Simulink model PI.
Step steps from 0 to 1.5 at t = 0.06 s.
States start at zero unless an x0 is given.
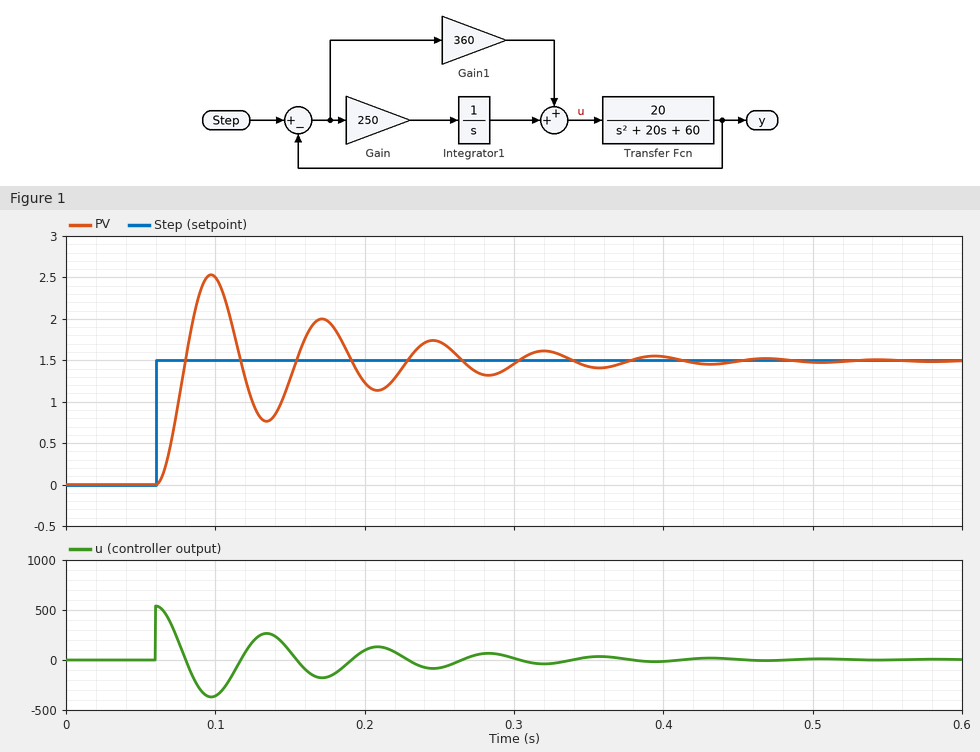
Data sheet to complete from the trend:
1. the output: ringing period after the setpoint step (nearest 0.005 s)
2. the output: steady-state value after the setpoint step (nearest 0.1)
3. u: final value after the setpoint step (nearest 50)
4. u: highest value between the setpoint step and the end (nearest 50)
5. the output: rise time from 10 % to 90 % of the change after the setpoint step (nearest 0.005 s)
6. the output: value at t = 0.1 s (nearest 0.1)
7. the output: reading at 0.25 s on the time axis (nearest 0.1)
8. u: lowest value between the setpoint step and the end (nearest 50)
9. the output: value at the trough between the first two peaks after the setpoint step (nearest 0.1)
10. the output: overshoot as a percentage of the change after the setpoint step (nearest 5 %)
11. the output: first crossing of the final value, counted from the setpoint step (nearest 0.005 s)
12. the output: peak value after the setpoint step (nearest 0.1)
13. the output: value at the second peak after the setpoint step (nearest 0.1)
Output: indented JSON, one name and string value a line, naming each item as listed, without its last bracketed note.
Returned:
{
  "the output: ringing period after the setpoint step": "0.075 s",
  "the output: steady-state value after the setpoint step": "1.5",
  "u: final value after the setpoint step": "0",
  "u: highest value between the setpoint step and the end": "550",
  "the output: rise time from 10 % to 90 % of the change after the setpoint step": "0.015 s",
  "the output: value at t = 0.1 s": "2.5",
  "the output: reading at 0.25 s on the time axis": "1.7",
  "u: lowest value between the setpoint step and the end": "-350",
  "the output: value at the trough between the first two peaks after the setpoint step": "0.8",
  "the output: overshoot as a percentage of the change after the setpoint step": "70 %",
  "the output: first crossing of the final value, counted from the setpoint step": "0.020 s",
  "the output: peak value after the setpoint step": "2.5",
  "the output: value at the second peak after the setpoint step": "2.0"
}
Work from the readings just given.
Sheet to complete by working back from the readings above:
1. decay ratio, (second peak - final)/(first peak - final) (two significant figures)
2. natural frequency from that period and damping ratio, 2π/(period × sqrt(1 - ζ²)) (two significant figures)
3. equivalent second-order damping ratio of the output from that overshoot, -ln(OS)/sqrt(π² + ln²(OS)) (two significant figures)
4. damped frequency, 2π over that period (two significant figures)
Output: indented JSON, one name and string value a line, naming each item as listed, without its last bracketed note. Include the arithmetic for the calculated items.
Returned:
{
  "decay ratio, (second peak - final)/(first peak - final)": "(2 - 1.5) / (2.5 - 1.5) = 0.50",
  "natural frequency from that period and damping ratio, 2π/(period × sqrt(1 - ζ²))": "2π / (0.075 × sqrt(1 - 0.11²)) = 84 rad/s",
  "equivalent second-order damping ratio of the output from that overshoot, -ln(OS)/sqrt(π² + ln²(OS))": "ln(0.7) = -0.357; 0.357 / sqrt(9.870 + 0.127) = 0.11",
  "damped frequency, 2π over that period": "2π / 0.075 = 84 rad/s"
}
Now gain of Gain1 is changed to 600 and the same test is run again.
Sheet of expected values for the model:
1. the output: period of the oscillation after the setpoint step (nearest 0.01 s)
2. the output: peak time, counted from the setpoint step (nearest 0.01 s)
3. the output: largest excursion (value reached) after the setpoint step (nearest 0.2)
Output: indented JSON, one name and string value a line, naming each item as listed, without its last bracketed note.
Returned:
{
  "the output: period of the oscillation after the setpoint step": "0.06 s",
  "the output: peak time, counted from the setpoint step": "0.03 s",
  "the output: largest excursion (value reached) after the setpoint step": "2.6"
}
